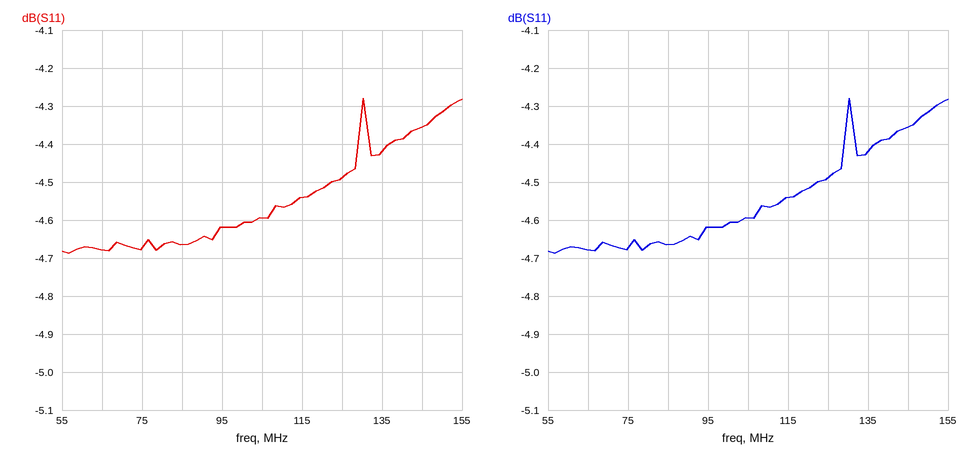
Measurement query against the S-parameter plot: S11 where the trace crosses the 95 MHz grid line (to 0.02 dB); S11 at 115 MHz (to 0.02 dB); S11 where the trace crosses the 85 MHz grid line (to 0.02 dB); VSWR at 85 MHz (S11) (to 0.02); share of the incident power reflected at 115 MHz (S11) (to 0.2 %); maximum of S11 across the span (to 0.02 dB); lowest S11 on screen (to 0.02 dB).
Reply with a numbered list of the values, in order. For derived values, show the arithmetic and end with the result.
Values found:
1. -4.62 dB
2. -4.54 dB
3. -4.66 dB
4. |Γ| = 10^(-4.66/20) = 0.5848; VSWR = (1 + 0.5848)/(1 − 0.5848) ≈ 3.82
5. 10^(-4.54/10) ≈ 35.2 %
6. -4.28 dB
7. -4.68 dB
